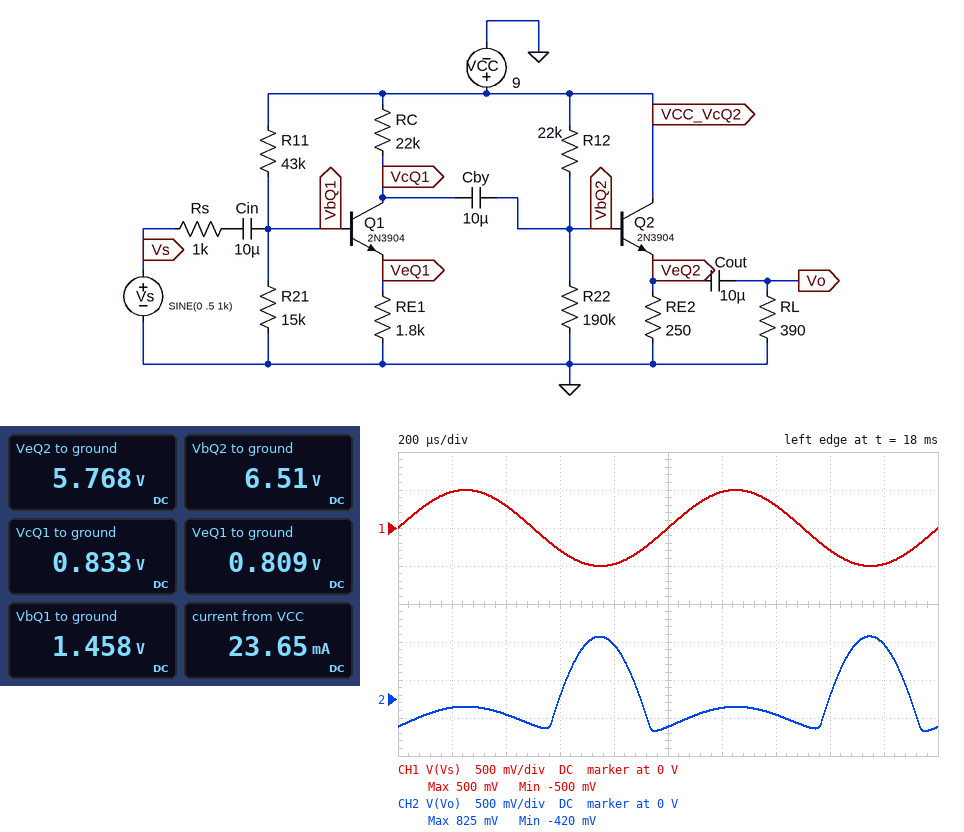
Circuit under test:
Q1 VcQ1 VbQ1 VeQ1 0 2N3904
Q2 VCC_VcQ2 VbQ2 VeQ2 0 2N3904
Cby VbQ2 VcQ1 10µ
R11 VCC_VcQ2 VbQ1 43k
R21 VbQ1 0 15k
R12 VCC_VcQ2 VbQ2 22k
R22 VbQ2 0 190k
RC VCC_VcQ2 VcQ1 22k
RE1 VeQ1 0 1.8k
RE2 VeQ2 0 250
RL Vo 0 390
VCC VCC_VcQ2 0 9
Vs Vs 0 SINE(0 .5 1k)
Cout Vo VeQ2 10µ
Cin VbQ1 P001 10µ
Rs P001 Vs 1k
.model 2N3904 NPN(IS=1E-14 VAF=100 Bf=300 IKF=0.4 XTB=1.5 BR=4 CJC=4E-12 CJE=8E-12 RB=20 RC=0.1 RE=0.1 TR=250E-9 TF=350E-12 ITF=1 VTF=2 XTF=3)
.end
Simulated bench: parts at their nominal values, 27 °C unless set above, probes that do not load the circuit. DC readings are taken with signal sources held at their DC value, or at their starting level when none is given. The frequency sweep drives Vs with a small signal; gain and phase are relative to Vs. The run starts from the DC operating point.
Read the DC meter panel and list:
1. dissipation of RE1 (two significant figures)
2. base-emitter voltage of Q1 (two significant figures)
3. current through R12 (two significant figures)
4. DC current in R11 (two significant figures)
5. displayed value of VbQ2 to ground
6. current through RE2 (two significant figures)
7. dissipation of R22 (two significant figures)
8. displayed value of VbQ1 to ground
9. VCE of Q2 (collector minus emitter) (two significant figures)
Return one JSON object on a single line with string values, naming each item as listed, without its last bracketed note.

{"dissipation of RE1": "360 µW", "base-emitter voltage of Q1": "650 mV", "current through R12": "110 µA", "DC current in R11": "180 µA", "displayed value of VbQ2 to ground": "6.51 V", "current through RE2": "23 mA", "dissipation of R22": "220 µW", "displayed value of VbQ1 to ground": "1.458 V", "VCE of Q2 (collector minus emitter)": "3.2 V"}
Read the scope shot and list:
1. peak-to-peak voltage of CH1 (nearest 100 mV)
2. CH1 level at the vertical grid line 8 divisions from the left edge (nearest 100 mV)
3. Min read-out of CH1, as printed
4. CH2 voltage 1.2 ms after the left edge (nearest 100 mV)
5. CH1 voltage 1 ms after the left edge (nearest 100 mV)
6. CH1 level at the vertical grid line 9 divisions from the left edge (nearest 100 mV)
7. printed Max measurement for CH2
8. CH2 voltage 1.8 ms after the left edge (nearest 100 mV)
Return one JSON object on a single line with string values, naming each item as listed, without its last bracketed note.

{"peak-to-peak voltage of CH1": "1.0 V", "CH1 level at the vertical grid line 8 divisions from the left edge": "-300 mV", "Min read-out of CH1, as printed": "-500 mV", "CH2 voltage 1.2 ms after the left edge": "-100 mV", "CH1 voltage 1 ms after the left edge": "0 V", "CH1 level at the vertical grid line 9 divisions from the left edge": "-500 mV", "printed Max measurement for CH2": "825 mV", "CH2 voltage 1.8 ms after the left edge": "700 mV"}
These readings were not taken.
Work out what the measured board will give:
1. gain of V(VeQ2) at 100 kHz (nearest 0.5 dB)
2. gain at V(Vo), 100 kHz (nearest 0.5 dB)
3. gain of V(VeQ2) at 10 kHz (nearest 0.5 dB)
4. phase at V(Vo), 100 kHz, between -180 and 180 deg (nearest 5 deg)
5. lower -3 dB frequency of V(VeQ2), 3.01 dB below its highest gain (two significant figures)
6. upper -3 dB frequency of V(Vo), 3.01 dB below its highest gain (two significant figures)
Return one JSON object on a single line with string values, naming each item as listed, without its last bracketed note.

{"gain of V(VeQ2) at 100 kHz": "-6.0 dB", "gain at V(Vo), 100 kHz": "-6.0 dB", "gain of V(VeQ2) at 10 kHz": "-6.5 dB", "phase at V(Vo), 100 kHz, between -180 and 180 deg": "5 deg", "lower -3 dB frequency of V(VeQ2), 3.01 dB below its highest gain": "10 Hz", "upper -3 dB frequency of V(Vo), 3.01 dB below its highest gain": "52 MHz"}
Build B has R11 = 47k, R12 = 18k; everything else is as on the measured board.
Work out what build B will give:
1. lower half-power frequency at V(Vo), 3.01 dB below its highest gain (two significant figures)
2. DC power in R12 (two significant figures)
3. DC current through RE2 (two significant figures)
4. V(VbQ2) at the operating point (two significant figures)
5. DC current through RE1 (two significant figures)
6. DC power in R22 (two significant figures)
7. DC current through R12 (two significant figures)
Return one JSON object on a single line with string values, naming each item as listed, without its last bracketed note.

{"lower half-power frequency at V(Vo), 3.01 dB below its highest gain": "79 Hz", "DC power in R12": "260 µW", "DC current through RE2": "24 mA", "V(VbQ2) at the operating point": "6.8 V", "DC current through RE1": "440 µA", "DC power in R22": "250 µW", "DC current through R12": "120 µA"}
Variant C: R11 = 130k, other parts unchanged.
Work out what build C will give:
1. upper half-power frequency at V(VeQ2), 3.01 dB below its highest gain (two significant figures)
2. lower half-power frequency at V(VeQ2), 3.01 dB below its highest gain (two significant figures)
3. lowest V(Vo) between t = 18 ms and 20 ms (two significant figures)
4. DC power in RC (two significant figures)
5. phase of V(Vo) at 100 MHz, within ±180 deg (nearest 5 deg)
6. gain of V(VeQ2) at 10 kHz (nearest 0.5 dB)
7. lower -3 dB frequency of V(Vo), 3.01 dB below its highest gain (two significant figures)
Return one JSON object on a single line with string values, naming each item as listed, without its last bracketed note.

{"upper half-power frequency at V(VeQ2), 3.01 dB below its highest gain": "2.0 MHz", "lower half-power frequency at V(VeQ2), 3.01 dB below its highest gain": "1.2 Hz", "lowest V(Vo) between t = 18 ms and 20 ms": "-1.9 V", "DC power in RC": "670 µW", "phase of V(Vo) at 100 MHz, within ±180 deg": "-25 deg", "gain of V(VeQ2) at 10 kHz": "12.0 dB", "lower -3 dB frequency of V(Vo), 3.01 dB below its highest gain": "38 Hz"}
